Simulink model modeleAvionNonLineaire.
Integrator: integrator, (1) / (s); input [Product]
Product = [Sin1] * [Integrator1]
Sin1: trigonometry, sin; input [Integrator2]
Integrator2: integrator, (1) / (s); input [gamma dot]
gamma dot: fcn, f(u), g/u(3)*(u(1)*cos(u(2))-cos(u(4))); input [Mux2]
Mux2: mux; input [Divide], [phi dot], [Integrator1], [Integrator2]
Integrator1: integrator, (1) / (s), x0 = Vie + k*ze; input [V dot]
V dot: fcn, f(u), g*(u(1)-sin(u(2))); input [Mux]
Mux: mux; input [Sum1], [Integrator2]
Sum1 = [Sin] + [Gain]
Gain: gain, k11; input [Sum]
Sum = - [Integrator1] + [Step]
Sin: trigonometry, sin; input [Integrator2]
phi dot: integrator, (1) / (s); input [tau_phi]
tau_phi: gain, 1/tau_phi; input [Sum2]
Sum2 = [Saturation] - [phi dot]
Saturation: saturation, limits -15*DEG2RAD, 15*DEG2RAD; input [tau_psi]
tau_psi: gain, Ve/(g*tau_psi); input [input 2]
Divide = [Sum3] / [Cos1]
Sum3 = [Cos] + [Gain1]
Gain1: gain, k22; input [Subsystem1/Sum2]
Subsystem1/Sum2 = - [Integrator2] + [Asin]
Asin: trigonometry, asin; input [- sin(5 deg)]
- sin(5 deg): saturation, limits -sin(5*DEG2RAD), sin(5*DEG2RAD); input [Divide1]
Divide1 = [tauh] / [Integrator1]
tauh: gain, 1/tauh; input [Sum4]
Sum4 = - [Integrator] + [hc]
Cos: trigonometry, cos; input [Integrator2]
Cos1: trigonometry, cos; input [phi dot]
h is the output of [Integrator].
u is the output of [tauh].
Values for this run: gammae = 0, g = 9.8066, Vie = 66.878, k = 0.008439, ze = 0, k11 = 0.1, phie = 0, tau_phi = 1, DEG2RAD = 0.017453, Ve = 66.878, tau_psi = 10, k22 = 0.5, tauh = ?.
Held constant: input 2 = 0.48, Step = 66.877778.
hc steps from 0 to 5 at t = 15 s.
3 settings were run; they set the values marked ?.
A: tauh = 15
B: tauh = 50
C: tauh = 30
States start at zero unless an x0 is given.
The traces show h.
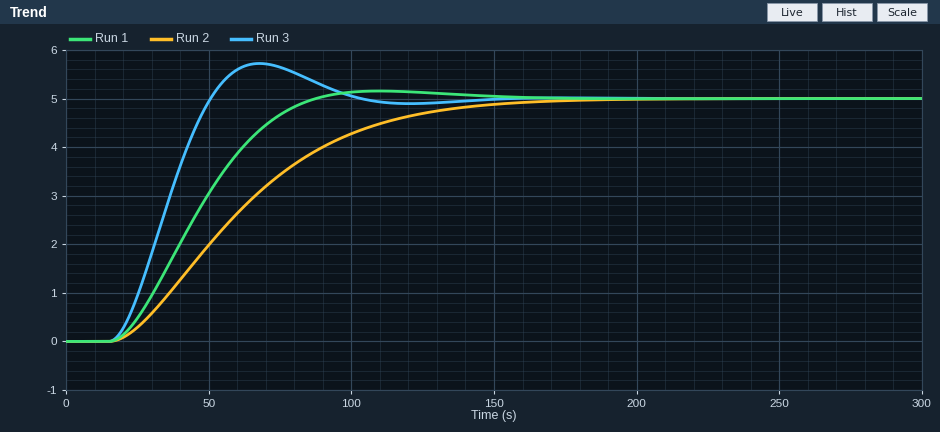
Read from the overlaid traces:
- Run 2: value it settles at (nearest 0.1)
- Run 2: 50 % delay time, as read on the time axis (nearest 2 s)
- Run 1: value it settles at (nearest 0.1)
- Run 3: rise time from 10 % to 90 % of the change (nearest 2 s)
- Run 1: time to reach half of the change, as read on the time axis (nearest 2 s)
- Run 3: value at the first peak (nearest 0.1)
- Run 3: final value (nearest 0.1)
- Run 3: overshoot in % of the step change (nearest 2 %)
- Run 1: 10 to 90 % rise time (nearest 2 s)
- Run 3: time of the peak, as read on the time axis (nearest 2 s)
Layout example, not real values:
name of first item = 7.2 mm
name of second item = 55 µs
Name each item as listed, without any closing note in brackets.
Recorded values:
Run 2: value it settles at = 5.0
Run 2: 50 % delay time, as read on the time axis = 58 s
Run 1: value it settles at = 5.0
Run 3: rise time from 10 % to 90 % of the change = 24 s
Run 1: time to reach half of the change, as read on the time axis = 44 s
Run 3: value at the first peak = 5.7
Run 3: final value = 5.0
Run 3: overshoot in % of the step change = 14 %
Run 1: 10 to 90 % rise time = 46 s
Run 3: time of the peak, as read on the time axis = 68 s
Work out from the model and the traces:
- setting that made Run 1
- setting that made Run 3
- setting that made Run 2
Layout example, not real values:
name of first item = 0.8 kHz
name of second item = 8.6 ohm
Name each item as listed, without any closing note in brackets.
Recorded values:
setting that made Run 1 = C
setting that made Run 3 = A
setting that made Run 2 = B
